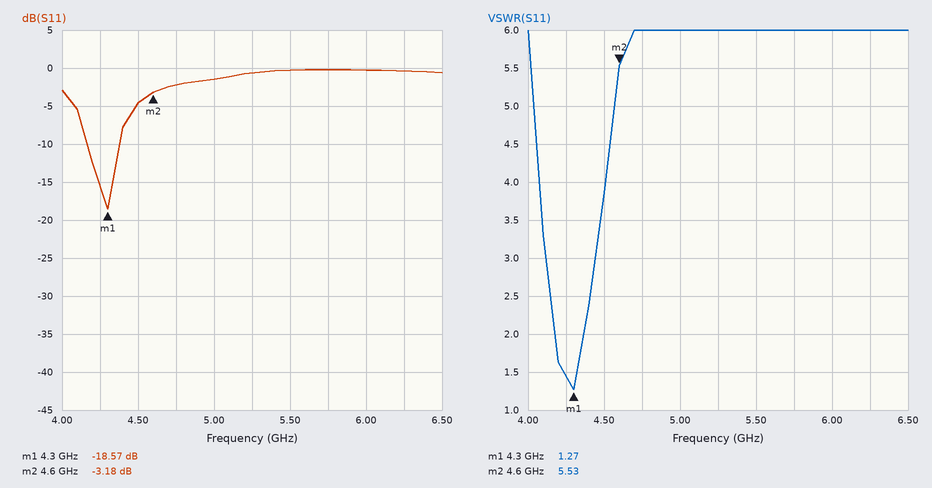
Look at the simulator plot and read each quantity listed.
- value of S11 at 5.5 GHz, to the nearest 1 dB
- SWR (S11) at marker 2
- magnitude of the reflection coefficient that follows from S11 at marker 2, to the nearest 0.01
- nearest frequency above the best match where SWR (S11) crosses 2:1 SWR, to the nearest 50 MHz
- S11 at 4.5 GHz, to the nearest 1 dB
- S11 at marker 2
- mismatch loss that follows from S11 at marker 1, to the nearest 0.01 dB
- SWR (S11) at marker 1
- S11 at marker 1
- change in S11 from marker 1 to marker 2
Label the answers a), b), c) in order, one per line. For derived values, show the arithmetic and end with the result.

a) 0 dB
b) 5.53
c) 10^(-3.18/20) ≈ 0.69
d) 4.35 GHz
e) -5 dB
f) -3.18 dB
g) −10 log10(1 − 10^(-18.57/10)) ≈ 0.06 dB
h) 1.27
i) -18.57 dB
j) -3.18 − (-18.57) = 15.39 dB
